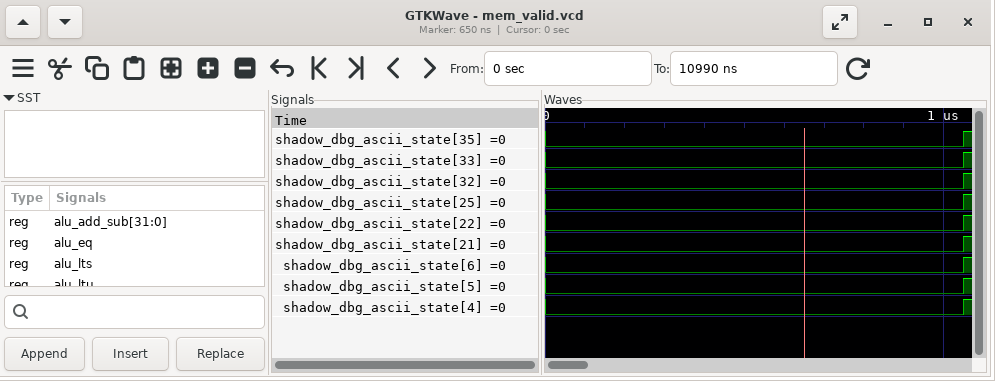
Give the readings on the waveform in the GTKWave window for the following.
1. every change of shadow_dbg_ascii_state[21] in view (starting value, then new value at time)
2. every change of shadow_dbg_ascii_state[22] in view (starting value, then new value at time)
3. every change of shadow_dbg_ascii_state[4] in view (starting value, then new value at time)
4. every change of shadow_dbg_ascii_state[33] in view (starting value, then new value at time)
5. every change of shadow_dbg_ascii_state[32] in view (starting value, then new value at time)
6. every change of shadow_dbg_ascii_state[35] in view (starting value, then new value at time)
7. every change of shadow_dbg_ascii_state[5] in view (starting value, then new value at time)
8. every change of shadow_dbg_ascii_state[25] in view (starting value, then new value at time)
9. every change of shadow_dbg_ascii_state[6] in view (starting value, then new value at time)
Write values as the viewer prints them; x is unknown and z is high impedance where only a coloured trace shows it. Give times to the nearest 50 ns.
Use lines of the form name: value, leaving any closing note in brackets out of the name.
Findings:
every change of shadow_dbg_ascii_state[21] in view: 0, 1 at 1050 ns
every change of shadow_dbg_ascii_state[22] in view: 0, 1 at 1050 ns
every change of shadow_dbg_ascii_state[4] in view: 0, 1 at 1050 ns
every change of shadow_dbg_ascii_state[33] in view: 0, 1 at 1050 ns
every change of shadow_dbg_ascii_state[32] in view: 0, 1 at 1050 ns
every change of shadow_dbg_ascii_state[35] in view: 0, 1 at 1050 ns
every change of shadow_dbg_ascii_state[5] in view: 0, 1 at 1050 ns
every change of shadow_dbg_ascii_state[25] in view: 0, 1 at 1050 ns
every change of shadow_dbg_ascii_state[6] in view: 0, 1 at 1050 ns
